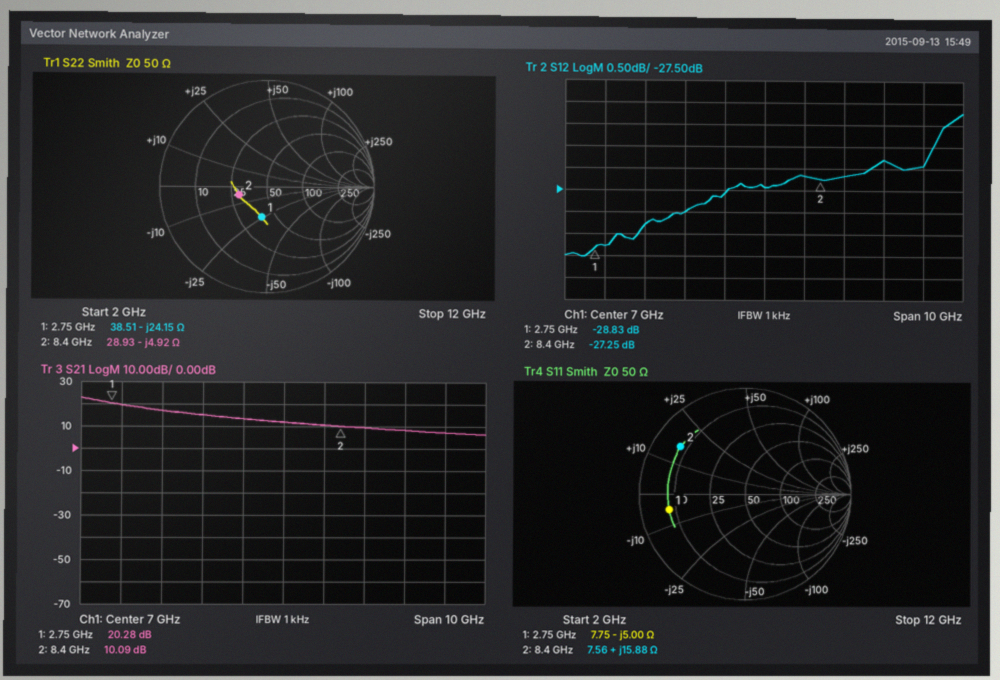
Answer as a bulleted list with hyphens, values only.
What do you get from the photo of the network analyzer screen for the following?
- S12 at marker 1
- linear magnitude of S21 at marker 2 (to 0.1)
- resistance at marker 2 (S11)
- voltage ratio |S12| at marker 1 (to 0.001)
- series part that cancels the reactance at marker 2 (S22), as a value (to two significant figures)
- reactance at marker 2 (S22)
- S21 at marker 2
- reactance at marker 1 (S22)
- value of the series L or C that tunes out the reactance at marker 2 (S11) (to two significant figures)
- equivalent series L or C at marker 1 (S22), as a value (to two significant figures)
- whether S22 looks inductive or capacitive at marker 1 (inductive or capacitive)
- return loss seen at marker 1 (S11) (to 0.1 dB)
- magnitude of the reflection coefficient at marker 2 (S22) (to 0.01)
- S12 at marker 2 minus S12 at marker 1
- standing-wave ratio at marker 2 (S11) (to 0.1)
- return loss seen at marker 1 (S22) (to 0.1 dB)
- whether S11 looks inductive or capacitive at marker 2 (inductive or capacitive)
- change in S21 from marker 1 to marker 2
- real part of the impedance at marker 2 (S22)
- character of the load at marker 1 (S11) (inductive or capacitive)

- -28.83 dB
- 3.2
- 7.56 Ω
- 0.036
- 93 pH
- -4.92 Ω
- 10.09 dB
- -24.15 Ω
- 1.2 pF
- 2.4 pF
- capacitive
- 2.7 dB
- 0.27
- 1.58 dB
- 7.3
- 10.7 dB
- inductive
- -10.19 dB
- 28.93 Ω
- capacitive
